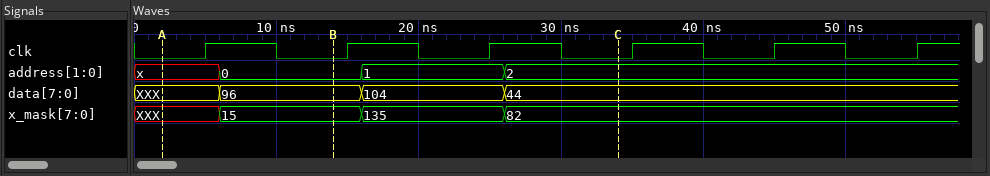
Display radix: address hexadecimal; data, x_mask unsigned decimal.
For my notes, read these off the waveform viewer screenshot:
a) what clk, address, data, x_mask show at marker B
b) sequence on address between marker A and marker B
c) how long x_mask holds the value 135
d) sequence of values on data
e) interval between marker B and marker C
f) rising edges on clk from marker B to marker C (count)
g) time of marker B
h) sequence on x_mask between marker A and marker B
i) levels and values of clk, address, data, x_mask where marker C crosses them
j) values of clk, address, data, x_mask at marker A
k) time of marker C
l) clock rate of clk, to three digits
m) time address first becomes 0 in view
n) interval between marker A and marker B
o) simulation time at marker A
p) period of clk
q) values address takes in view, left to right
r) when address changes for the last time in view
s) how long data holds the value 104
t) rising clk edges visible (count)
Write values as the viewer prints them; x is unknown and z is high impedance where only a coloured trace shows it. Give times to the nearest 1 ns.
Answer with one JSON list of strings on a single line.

["clk=0, address=0, data=96, x_mask=15", "x, 0", "10 ns", "XXX, 96, 104, 44", "20 ns", "2", "14 ns", "XXX, 15", "clk=0, address=2, data=44, x_mask=82", "clk=0, address=x, data=XXX, x_mask=XXX", "34 ns", "100 MHz", "6 ns", "12 ns", "2 ns", "10 ns", "x, 0, 1, 2", "26 ns", "10 ns", "6"]
